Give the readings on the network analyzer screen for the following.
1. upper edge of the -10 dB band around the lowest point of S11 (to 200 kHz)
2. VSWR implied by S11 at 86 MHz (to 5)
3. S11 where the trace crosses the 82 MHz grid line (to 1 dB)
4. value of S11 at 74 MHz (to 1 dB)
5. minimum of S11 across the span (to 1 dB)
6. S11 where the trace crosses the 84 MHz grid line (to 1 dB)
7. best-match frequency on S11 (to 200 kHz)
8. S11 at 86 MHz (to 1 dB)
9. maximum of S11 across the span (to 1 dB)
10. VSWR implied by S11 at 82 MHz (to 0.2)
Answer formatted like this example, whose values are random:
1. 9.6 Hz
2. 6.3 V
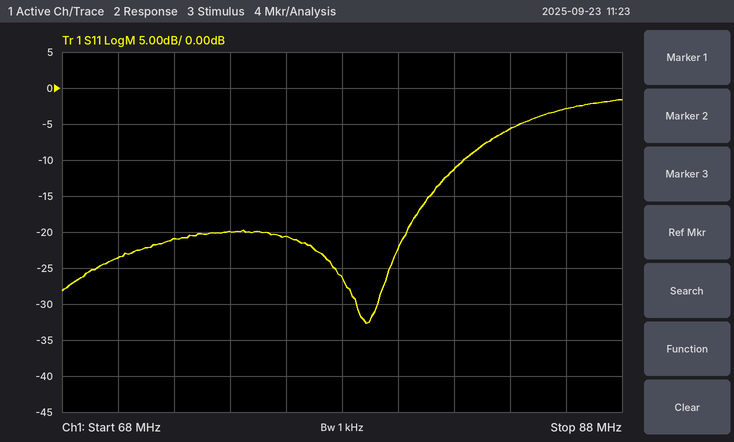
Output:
1. 82.4 MHz
2. 5
3. -11 dB
4. -20 dB
5. -33 dB
6. -6 dB
7. 78.8 MHz
8. -3 dB
9. -2 dB
10. 1.8
